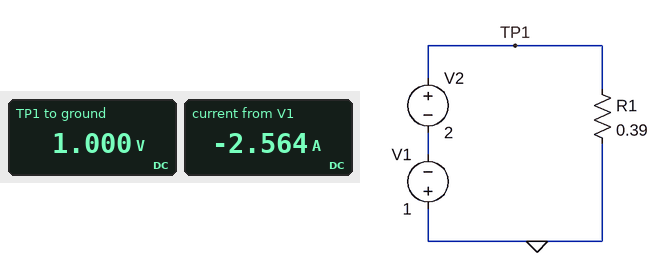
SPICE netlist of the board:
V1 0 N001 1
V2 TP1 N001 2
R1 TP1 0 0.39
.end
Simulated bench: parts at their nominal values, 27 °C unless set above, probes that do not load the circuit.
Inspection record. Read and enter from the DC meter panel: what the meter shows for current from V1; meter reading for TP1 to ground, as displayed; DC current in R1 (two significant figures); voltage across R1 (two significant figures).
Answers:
-2.564 A
1.000 V
2.6 A
1.0 V
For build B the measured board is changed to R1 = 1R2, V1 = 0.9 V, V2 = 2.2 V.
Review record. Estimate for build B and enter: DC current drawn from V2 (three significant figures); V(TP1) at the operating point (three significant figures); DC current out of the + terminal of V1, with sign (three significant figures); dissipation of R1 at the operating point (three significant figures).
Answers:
1.08 A
1.30 V
-1.08 A
1.41 W
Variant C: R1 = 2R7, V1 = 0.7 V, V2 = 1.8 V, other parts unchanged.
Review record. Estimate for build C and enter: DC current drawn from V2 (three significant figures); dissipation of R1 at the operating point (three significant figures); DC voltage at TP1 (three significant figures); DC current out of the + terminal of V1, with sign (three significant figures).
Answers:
407 mA
448 mW
1.10 V
-407 mA
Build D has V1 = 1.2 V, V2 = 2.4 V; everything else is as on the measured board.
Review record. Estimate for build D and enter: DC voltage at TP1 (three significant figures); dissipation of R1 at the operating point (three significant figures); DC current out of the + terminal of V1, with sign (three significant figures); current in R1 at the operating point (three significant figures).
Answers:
1.20 V
3.69 W
-3.08 A
3.08 A
